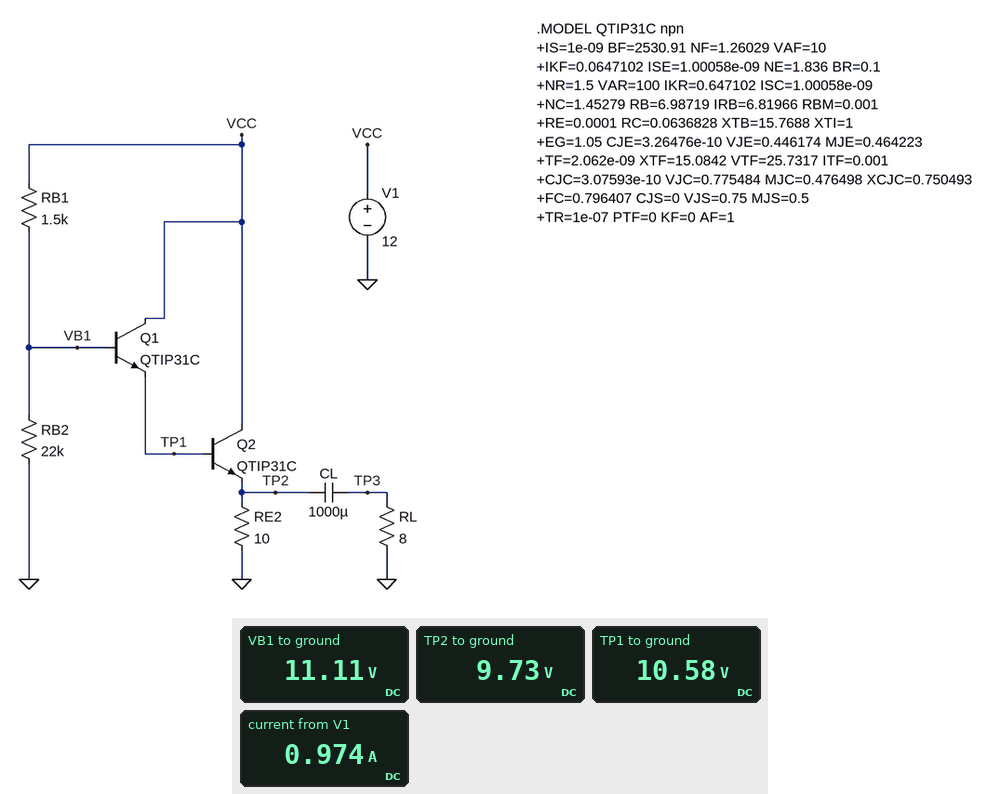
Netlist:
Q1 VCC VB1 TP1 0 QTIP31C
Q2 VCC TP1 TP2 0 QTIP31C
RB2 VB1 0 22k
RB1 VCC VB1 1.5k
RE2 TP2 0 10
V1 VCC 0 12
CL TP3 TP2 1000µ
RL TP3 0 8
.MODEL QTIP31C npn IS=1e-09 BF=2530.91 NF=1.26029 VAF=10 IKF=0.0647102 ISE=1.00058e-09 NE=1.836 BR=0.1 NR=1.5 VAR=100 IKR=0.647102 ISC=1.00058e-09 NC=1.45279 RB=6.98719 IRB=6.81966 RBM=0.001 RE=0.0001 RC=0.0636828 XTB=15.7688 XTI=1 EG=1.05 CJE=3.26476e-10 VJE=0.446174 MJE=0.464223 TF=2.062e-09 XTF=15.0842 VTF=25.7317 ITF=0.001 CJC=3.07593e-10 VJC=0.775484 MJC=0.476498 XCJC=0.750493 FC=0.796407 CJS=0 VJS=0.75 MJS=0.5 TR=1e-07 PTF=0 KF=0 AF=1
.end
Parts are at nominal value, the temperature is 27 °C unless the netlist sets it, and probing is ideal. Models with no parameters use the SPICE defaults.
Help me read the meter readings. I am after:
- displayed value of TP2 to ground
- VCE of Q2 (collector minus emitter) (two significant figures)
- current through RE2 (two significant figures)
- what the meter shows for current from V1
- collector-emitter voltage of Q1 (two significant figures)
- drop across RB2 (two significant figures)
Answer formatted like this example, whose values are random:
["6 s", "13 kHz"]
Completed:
["9.73 V", "2.3 V", "970 mA", "0.974 A", "1.4 V", "11 V"]
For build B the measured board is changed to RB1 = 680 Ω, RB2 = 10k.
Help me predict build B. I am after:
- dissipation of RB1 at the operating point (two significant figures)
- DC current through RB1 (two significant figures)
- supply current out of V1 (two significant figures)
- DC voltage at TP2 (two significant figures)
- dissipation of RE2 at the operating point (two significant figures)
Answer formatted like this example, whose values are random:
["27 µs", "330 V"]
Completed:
["990 µW", "1.2 mA", "980 mA", "9.8 V", "9.6 W"]
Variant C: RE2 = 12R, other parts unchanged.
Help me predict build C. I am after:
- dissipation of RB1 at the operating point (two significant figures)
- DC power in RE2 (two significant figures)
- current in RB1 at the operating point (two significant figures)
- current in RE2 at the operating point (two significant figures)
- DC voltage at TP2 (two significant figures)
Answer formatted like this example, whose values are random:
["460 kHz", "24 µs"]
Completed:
["500 µW", "8.0 W", "580 µA", "820 mA", "9.8 V"]
